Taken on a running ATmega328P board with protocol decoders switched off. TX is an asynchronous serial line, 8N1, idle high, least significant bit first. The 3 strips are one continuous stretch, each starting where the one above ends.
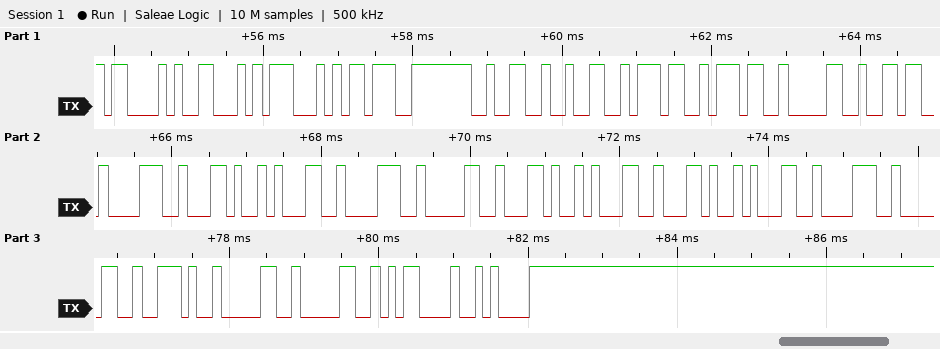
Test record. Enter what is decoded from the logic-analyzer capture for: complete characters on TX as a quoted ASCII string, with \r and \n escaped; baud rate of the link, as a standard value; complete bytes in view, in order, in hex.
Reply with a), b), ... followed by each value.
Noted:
a) "CFG;2277068,180,1,180.00\r\n"
b) 9600 baud
c) 43 46 47 3B 32 32 37 37 30 36 38 2C 31 38 30 2C 31 2C 31 38 30 2E 30 30 0D 0A
